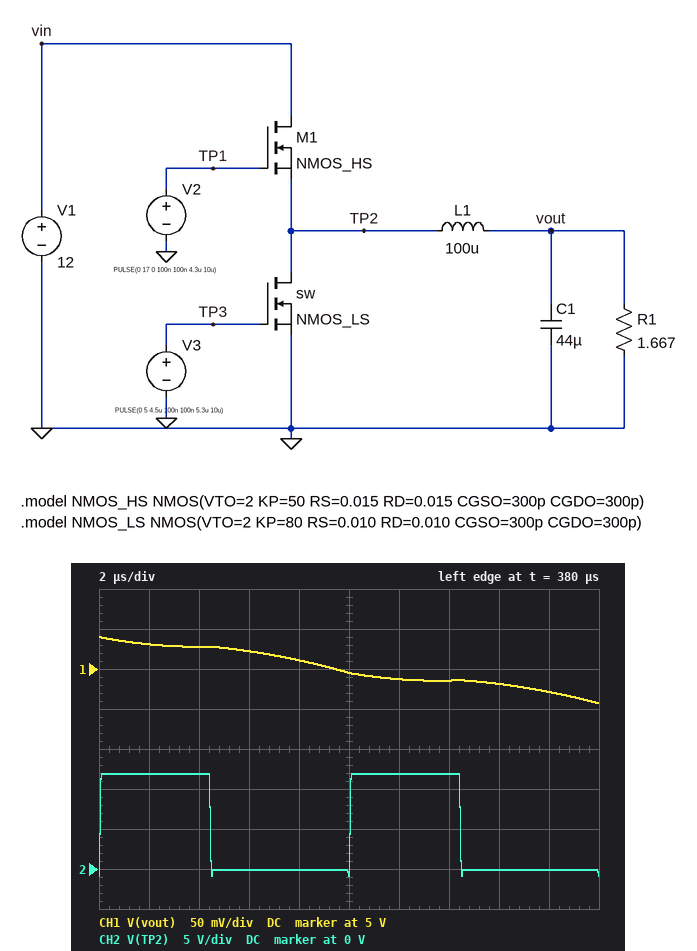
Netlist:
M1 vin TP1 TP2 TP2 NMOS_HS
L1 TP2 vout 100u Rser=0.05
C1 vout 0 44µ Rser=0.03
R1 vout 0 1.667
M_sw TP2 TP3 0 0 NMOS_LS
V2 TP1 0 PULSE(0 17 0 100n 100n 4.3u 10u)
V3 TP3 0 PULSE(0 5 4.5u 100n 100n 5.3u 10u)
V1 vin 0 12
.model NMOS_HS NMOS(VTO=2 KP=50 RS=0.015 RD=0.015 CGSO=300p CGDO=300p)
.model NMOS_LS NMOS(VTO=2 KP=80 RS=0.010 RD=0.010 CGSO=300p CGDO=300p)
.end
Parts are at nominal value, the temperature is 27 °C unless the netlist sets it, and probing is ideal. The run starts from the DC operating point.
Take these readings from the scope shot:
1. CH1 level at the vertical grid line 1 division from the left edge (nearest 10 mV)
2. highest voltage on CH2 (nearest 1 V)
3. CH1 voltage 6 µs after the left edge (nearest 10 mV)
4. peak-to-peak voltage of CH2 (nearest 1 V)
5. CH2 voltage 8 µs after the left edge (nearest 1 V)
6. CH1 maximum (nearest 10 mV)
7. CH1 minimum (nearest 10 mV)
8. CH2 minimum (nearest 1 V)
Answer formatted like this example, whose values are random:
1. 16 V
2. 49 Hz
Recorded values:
1. 5.03 V
2. 12 V
3. 5.02 V
4. 13 V
5. 0 V
6. 5.04 V
7. 4.96 V
8. -1 V
